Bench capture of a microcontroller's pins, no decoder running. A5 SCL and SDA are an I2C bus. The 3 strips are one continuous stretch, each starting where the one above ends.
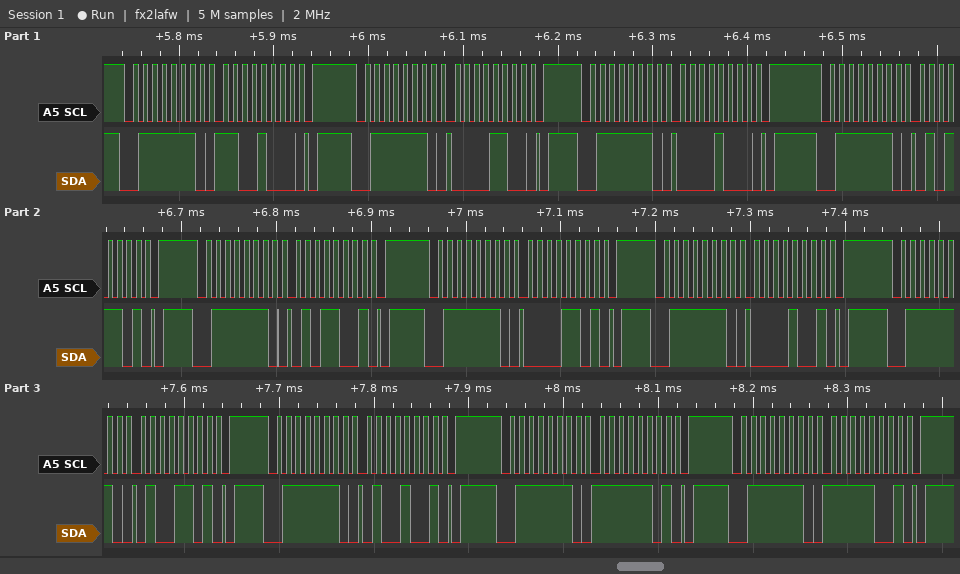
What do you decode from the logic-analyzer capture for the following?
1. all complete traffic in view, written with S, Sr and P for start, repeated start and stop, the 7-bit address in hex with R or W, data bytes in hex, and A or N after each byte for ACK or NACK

S 3FW A C8 A P S 3FW A 0C A P S 3FW A 08 A P S 3FW A 5D A P S 3FW A 59 A P S 3FW A 0D A P S 3FW A 09 A P S 3FW A 4D A P S 3FW A 49 A P S 3FW A FD A P S 3FW A F9 A P
